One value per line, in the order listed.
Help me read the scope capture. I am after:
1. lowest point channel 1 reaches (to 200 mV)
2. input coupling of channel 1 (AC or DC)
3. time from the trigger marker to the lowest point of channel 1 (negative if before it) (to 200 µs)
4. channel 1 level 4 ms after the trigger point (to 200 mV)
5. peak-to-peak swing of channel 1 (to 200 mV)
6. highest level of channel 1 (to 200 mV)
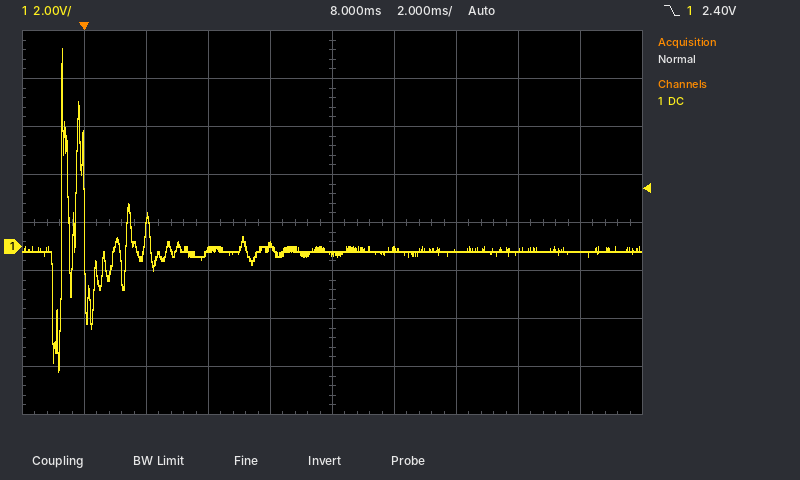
-5.2 V
DC
-800 µs
-200 mV
13.4 V
8.2 V
